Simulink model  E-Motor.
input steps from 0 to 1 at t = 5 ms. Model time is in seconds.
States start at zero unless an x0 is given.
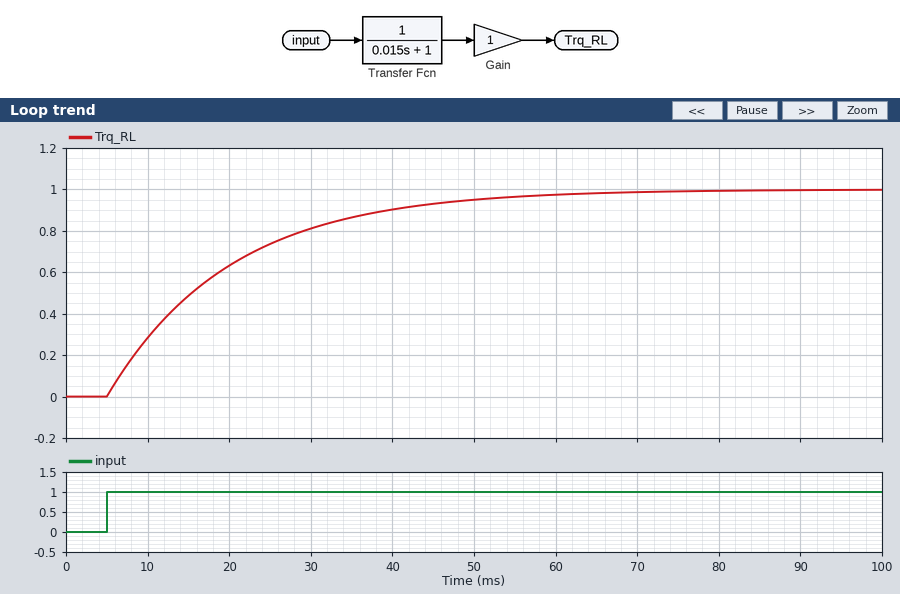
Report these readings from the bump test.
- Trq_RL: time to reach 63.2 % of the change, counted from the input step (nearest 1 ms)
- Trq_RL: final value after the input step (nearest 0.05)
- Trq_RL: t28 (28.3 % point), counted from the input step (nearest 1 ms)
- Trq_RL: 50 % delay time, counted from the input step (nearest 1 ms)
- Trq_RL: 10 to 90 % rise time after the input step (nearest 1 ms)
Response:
15 ms
1.00
5 ms
10 ms
33 ms
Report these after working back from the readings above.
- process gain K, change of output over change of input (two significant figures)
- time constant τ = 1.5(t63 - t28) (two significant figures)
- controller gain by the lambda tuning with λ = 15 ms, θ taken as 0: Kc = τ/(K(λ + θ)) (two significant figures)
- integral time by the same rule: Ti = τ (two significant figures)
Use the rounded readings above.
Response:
1.0
15 ms
1.0
15 ms
